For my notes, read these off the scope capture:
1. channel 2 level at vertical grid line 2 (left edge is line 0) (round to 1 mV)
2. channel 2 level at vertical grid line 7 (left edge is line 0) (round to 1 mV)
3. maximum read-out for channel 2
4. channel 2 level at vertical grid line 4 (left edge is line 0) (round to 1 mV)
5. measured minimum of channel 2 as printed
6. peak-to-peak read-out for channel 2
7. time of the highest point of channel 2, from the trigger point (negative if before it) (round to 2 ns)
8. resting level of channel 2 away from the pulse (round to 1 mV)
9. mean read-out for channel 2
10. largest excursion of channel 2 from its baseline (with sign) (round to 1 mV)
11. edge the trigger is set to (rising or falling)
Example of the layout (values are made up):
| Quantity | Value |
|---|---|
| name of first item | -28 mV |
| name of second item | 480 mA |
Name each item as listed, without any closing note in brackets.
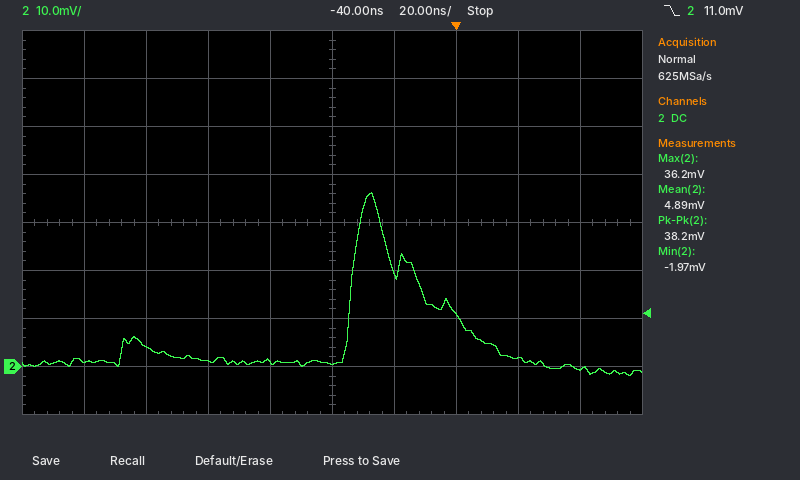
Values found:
| Quantity | Value |
|---|---|
| channel 2 level at vertical grid line 2 (left edge is line 0) | 4 mV |
| channel 2 level at vertical grid line 7 (left edge is line 0) | 11 mV |
| maximum read-out for channel 2 | 36.2 mV |
| channel 2 level at vertical grid line 4 (left edge is line 0) | 1 mV |
| measured minimum of channel 2 as printed | -1.97 mV |
| peak-to-peak read-out for channel 2 | 38.2 mV |
| time of the highest point of channel 2, from the trigger point (negative if before it) | -28 ns |
| resting level of channel 2 away from the pulse | 1 mV |
| mean read-out for channel 2 | 4.89 mV |
| largest excursion of channel 2 from its baseline (with sign) | +35 mV |
| edge the trigger is set to | falling |
